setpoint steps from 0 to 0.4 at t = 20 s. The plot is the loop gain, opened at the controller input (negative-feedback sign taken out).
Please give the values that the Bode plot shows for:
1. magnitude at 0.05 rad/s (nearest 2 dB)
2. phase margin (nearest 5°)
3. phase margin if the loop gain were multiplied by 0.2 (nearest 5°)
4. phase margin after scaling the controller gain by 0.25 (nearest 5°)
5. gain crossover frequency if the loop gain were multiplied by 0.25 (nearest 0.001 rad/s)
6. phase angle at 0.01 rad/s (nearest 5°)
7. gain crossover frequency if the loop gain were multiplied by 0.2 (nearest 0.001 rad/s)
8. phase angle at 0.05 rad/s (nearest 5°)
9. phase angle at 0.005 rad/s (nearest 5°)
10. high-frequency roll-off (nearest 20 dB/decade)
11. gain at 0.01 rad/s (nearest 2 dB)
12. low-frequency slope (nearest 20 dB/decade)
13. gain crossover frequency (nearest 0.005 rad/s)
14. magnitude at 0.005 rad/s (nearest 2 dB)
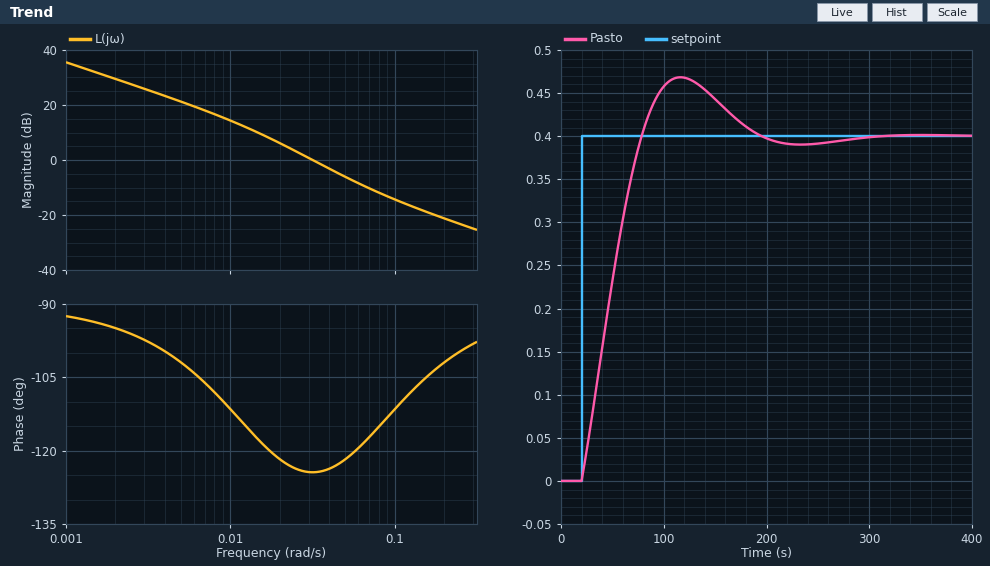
-6 dB
55°
70°
65°
0.012 rad/s
-110°
0.010 rad/s
-120°
-100°
-20 dB/decade
14 dB
-20 dB/decade
0.030 rad/s
22 dB
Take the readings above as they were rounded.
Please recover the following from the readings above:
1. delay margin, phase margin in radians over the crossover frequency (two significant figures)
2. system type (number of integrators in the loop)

32 s
1
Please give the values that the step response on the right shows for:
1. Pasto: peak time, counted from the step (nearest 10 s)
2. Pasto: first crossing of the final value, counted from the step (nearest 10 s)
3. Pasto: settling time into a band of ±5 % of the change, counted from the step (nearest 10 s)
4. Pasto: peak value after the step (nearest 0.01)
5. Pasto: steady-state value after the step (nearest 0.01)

100 s
60 s
150 s
0.47
0.40
